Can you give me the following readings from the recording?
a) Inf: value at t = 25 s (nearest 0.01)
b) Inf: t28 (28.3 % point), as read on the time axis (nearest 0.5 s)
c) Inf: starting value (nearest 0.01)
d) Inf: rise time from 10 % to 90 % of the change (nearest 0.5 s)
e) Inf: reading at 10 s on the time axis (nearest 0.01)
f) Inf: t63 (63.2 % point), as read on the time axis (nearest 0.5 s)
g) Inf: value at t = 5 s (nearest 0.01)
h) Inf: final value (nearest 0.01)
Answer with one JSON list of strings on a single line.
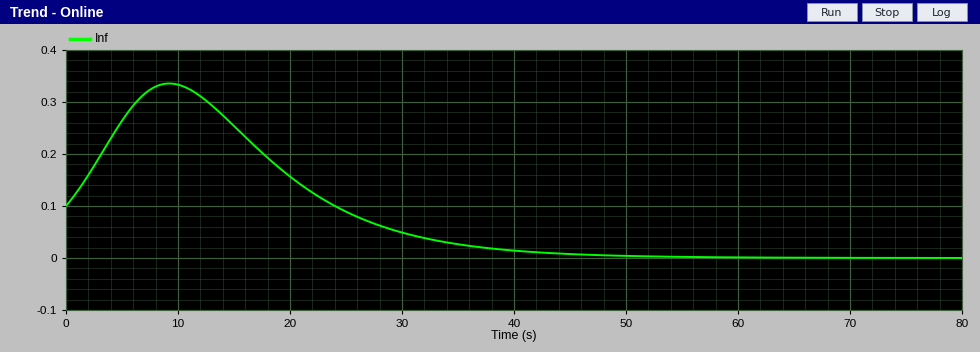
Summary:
["0.09", "27.0 s", "0.10", "18.0 s", "0.33", "32.5 s", "0.26", "0.00"]
